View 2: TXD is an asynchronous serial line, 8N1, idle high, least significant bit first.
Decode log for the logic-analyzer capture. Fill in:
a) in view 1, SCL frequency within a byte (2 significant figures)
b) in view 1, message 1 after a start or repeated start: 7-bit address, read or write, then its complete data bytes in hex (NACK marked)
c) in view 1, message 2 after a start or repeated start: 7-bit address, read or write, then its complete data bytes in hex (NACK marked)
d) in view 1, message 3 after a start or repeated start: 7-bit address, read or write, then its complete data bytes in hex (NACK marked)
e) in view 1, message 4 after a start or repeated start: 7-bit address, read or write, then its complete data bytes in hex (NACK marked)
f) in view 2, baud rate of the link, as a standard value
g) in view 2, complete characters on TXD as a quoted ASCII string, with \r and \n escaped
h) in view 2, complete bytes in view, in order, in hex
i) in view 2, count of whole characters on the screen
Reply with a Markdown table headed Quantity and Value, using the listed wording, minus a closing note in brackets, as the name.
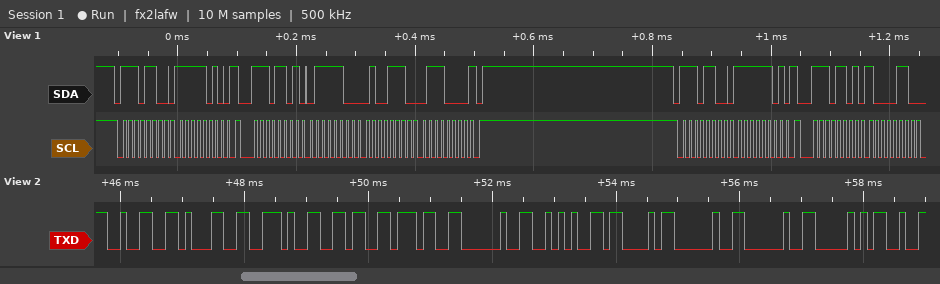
| Quantity | Value |
|---|---|
| in view 1, SCL frequency within a byte | 100 kHz |
| in view 1, message 1 after a start or repeated start: 7-bit address, read or write, then its complete data bytes in hex | 0x76 write: FA |
| in view 1, message 2 after a start or repeated start: 7-bit address, read or write, then its complete data bytes in hex | 0x76 read: 7C 4E 70 NACK |
| in view 1, message 3 after a start or repeated start: 7-bit address, read or write, then its complete data bytes in hex | 0x76 write: FD |
| in view 1, message 4 after a start or repeated start: 7-bit address, read or write, then its complete data bytes in hex | 0x76 read: 86 |
| in view 2, baud rate of the link, as a standard value | 9600 baud |
| in view 2, complete characters on TXD as a quoted ASCII string, with \r and \n escaped | "21.67 *C  P" |
| in view 2, complete bytes in view, in order, in hex | 32 31 2E 36 37 20 2A 43 20 20 50 |
| in view 2, count of whole characters on the screen | 11 |
